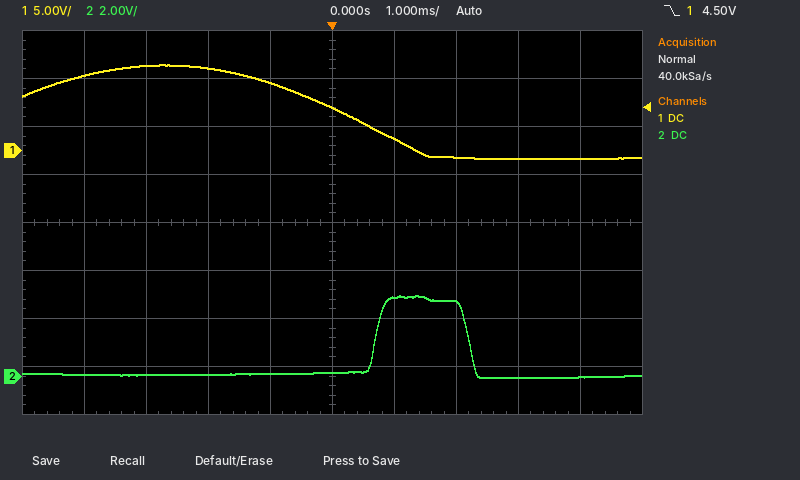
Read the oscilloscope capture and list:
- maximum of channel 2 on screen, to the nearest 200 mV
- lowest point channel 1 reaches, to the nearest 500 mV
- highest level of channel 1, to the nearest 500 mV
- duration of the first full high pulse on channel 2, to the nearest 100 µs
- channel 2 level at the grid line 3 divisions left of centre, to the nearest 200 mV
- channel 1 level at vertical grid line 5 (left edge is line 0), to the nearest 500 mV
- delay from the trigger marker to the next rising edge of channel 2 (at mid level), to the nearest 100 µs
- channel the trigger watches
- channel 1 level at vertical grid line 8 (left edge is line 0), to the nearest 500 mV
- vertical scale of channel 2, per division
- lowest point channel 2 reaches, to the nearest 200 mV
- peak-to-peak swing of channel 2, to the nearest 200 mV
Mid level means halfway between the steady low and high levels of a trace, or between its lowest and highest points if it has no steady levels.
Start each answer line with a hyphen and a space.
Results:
- 3.4 V
- -1.0 V
- 9.0 V
- 1.5 ms
- 0.0 V
- 4.5 V
- 700 µs
- channel 1
- -1.0 V
- 2 V
- 0.0 V
- 3.4 V
